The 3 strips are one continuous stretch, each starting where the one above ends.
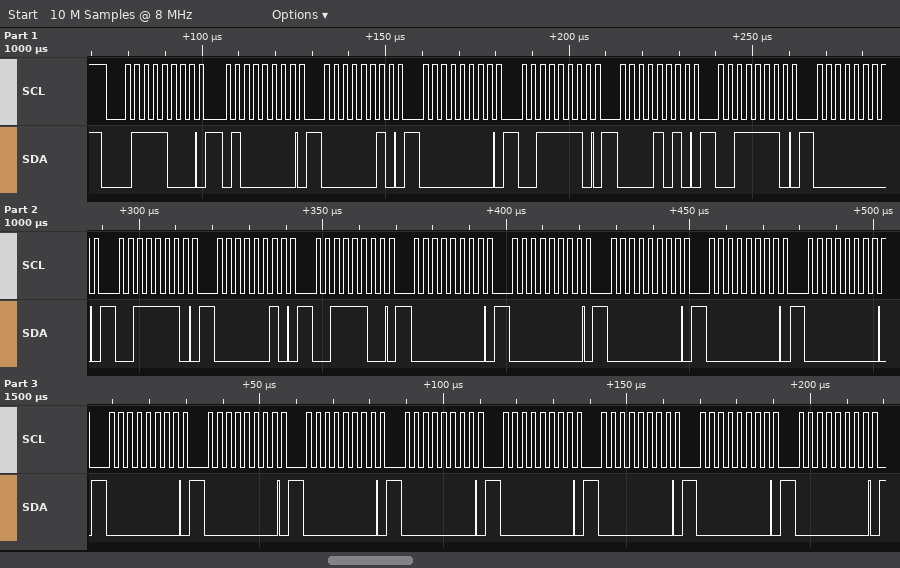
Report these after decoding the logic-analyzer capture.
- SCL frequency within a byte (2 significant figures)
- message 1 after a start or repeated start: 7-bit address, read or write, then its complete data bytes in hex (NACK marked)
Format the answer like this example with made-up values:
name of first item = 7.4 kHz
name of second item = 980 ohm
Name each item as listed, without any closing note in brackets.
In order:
SCL frequency within a byte = 400 kHz
message 1 after a start or repeated start: 7-bit address, read or write, then its complete data bytes in hex = 0x3C write: 40 02 00 3E 0A 3E 00 3E 02 3C 00 00 00 00 00 00 00 00 00 00 00 00 00
